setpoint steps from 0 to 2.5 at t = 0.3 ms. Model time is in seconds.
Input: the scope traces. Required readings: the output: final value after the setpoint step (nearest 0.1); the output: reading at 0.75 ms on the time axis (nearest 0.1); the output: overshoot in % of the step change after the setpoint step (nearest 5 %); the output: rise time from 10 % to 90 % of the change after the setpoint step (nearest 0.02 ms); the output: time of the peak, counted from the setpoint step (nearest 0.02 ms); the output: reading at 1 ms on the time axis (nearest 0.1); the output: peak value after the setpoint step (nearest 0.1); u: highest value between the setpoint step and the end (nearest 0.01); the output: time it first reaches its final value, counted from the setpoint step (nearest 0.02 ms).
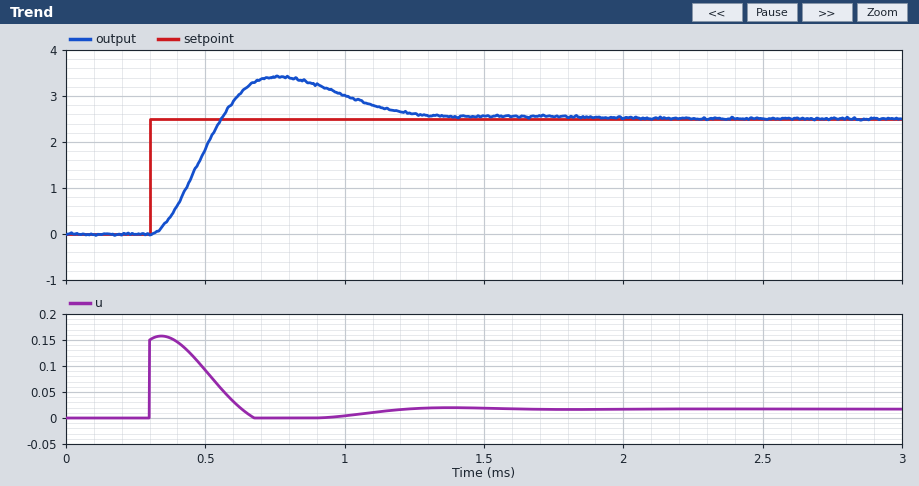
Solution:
2.5
3.4
35 %
0.18 ms
0.46 ms
3.0
3.4
0.16
0.26 ms
